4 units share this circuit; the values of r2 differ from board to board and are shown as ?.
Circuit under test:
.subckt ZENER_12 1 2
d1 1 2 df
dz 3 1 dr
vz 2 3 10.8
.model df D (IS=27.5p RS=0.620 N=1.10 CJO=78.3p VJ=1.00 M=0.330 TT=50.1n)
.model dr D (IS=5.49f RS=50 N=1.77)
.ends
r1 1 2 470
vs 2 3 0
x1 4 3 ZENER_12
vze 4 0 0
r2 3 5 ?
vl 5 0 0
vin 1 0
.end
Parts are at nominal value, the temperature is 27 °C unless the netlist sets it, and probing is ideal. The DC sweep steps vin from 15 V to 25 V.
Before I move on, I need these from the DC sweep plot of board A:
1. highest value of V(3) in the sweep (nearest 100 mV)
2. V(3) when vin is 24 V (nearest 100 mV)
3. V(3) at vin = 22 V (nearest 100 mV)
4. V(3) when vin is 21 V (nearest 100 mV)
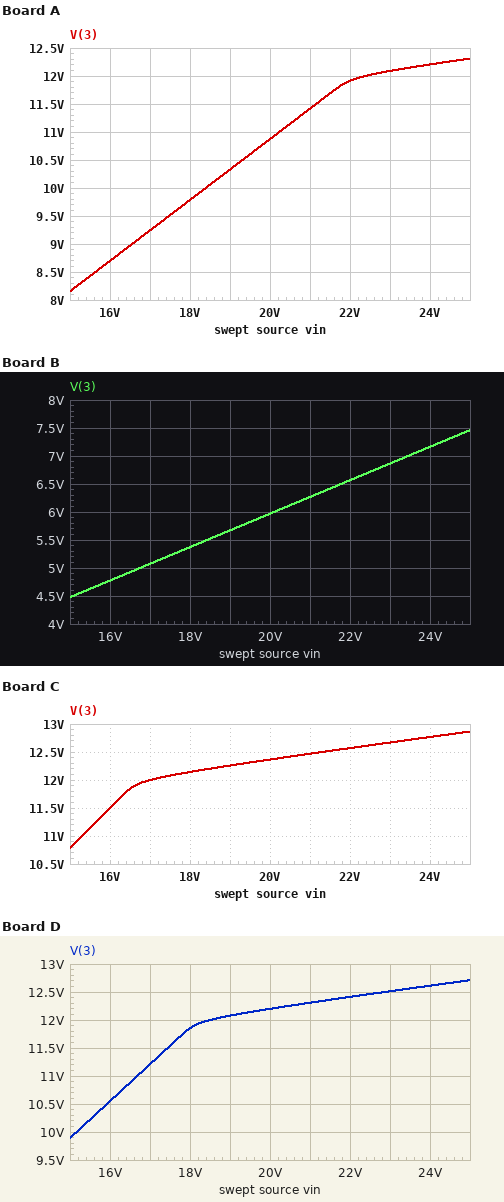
12.3 V
12.2 V
11.9 V
11.4 V
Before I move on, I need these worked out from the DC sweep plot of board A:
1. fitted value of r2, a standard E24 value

560 Ω
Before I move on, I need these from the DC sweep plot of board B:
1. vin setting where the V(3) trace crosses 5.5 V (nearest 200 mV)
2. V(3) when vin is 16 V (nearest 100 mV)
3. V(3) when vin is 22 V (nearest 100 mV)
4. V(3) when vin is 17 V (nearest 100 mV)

18.4 V
4.8 V
6.6 V
5.1 V
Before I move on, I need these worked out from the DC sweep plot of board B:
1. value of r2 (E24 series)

200 Ω
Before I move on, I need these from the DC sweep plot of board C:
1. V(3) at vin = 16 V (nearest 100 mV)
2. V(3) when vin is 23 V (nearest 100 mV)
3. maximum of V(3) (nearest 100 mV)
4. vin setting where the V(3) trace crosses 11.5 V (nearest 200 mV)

11.5 V
12.7 V
12.9 V
16.0 V
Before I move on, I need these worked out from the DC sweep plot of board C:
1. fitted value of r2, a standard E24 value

1.2 kΩ
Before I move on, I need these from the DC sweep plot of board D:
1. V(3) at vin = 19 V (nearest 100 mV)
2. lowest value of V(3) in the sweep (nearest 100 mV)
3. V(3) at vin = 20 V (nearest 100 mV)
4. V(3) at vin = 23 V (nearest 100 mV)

12.1 V
9.9 V
12.2 V
12.5 V
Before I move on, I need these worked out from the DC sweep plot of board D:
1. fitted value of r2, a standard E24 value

910 Ω
